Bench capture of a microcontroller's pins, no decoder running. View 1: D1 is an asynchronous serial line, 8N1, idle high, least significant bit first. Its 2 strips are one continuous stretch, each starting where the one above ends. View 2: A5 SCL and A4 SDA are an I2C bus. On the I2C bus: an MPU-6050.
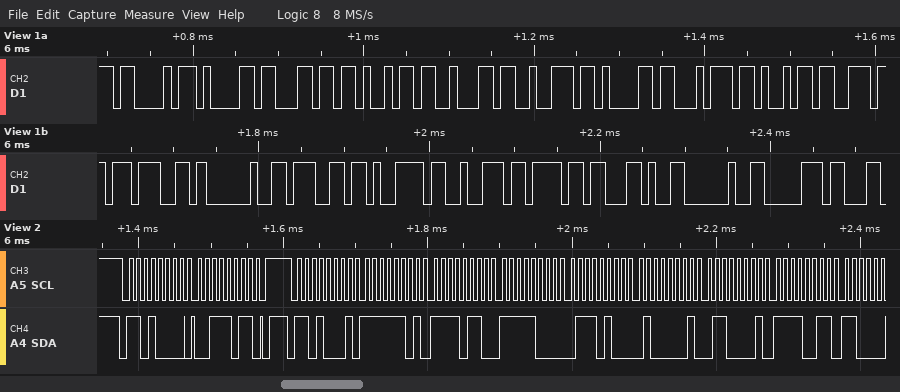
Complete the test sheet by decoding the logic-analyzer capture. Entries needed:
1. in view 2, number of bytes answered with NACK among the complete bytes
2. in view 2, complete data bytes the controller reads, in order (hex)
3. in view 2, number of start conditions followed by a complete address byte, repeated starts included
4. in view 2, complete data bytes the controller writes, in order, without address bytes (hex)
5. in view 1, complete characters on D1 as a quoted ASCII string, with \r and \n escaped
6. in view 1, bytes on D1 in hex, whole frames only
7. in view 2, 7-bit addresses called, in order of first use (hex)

0
FD F6 F8 74 41 61 F3
2
3B
"Calibrating gyro, p"
43 61 6C 69 62 72 61 74 69 6E 67 20 67 79 72 6F 2C 20 70
0x68
